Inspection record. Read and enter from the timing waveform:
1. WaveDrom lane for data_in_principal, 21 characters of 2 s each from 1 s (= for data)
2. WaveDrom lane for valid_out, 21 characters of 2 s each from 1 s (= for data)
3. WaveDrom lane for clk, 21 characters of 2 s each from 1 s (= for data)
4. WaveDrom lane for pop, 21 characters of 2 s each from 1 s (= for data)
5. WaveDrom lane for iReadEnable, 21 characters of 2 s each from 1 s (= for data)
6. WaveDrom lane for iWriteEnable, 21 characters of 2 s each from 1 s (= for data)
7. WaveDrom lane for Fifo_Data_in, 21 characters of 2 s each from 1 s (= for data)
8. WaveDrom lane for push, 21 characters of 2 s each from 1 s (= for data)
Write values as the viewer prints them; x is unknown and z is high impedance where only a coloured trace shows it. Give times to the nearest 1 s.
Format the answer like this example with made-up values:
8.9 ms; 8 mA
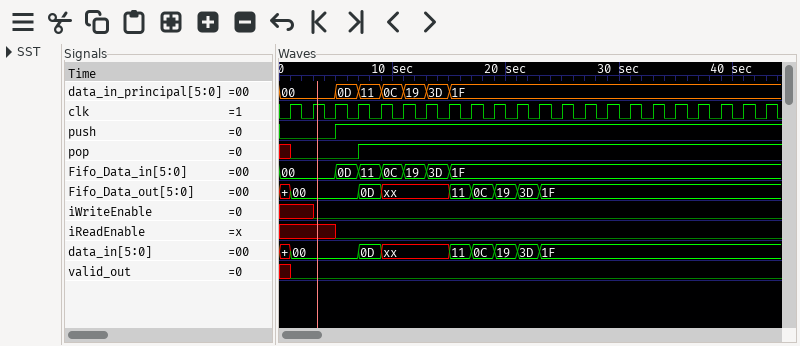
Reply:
{name: 'data_in_principal', wave: '=.======.............', data: '00 0D 11 0C 19 3D 1F'}; {name: 'valid_out', wave: '0....................'}; {name: 'clk', wave: 'p....................'}; {name: 'pop', wave: '0..1.................'}; {name: 'iReadEnable', wave: 'x.0..................'}; {name: 'iWriteEnable', wave: 'x0...................'}; {name: 'Fifo_Data_in', wave: '=.======.............', data: '00 0D 11 0C 19 3D 1F'}; {name: 'push', wave: '0.1..................'}
